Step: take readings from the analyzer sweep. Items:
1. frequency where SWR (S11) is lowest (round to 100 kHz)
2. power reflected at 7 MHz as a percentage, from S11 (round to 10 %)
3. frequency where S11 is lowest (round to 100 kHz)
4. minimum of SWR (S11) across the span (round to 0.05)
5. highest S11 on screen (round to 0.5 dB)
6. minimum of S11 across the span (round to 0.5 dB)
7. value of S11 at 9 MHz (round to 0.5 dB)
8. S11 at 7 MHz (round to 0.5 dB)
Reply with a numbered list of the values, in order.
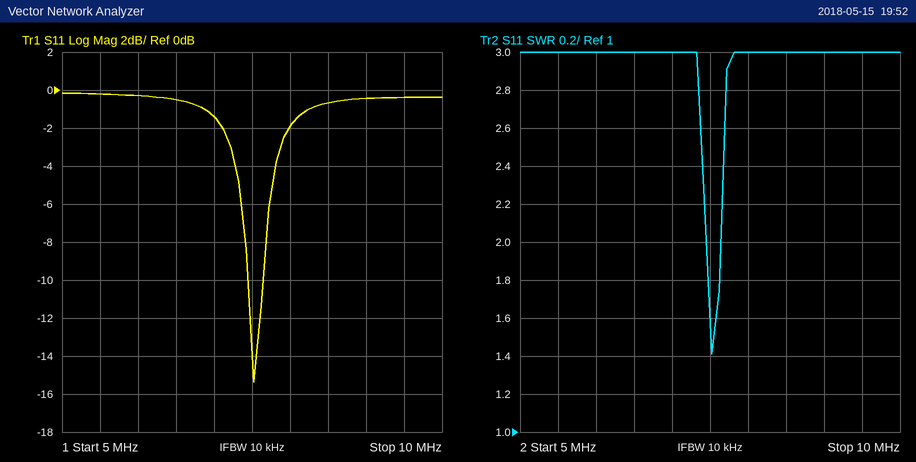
1. 7.5 MHz
2. 70 %
3. 7.5 MHz
4. 1.40
5. 0.0 dB
6. -15.5 dB
7. -0.5 dB
8. -1.5 dB
